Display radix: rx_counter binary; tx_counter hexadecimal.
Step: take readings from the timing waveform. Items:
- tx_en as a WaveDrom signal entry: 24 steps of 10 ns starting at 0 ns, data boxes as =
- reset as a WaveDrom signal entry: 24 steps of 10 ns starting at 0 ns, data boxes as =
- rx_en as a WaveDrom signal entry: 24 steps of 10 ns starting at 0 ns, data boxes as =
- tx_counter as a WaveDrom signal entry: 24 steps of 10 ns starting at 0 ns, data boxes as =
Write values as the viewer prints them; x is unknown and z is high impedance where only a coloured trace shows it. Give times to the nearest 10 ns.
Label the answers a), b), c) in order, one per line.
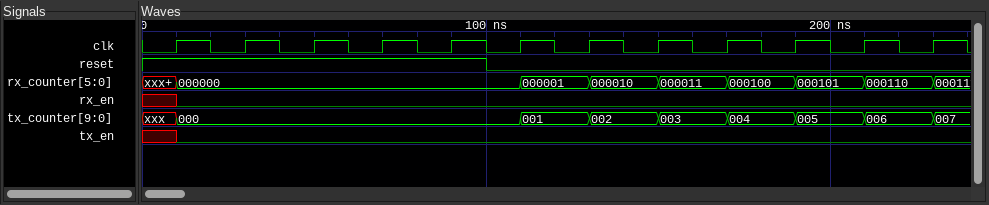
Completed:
a) {name: 'tx_en', wave: 'x0......................'}
b) {name: 'reset', wave: '1.........0.............'}
c) {name: 'rx_en', wave: 'x0......................'}
d) {name: 'tx_counter', wave: 'x=.........=.=.=.=.=.=.=', data: '000 001 002 003 004 005 006 007'}
